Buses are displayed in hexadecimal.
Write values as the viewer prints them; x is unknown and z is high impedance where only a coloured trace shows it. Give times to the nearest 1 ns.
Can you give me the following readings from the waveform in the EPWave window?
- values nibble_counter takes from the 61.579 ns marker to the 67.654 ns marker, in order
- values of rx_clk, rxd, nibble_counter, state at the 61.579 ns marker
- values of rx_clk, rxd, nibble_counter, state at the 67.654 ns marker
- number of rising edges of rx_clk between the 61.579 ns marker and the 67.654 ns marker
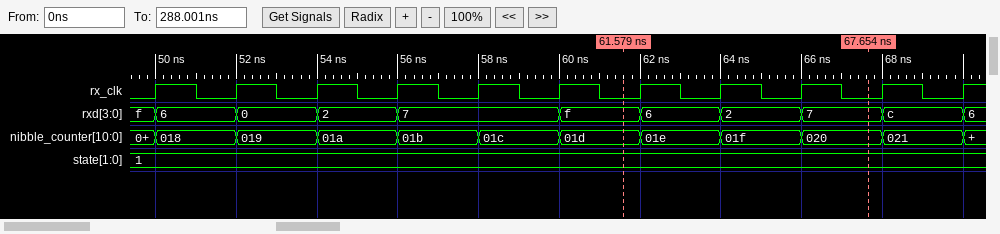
01d, 01e, 01f, 020
rx_clk=0, rxd=f, nibble_counter=01d, state=1
rx_clk=0, rxd=7, nibble_counter=020, state=1
3
